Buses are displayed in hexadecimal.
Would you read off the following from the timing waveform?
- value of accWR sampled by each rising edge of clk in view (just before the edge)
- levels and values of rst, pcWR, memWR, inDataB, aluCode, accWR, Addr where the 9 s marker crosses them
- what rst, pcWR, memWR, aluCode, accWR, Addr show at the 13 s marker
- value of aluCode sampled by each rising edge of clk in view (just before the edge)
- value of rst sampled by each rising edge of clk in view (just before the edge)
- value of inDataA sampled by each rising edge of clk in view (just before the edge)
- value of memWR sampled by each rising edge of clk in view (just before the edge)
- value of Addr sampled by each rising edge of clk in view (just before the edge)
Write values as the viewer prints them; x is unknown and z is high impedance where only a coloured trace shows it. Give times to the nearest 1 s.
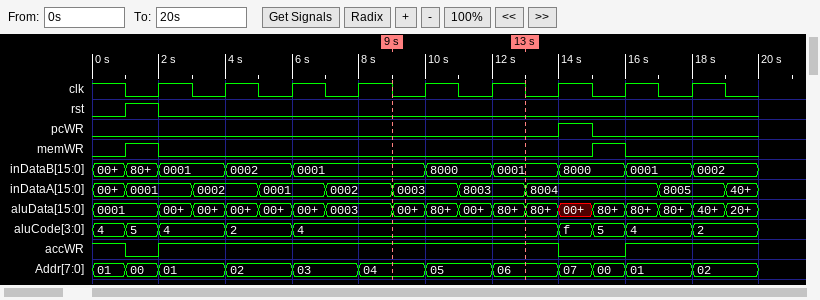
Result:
0 1 1 1 1 1 1 0 1
rst=0, pcWR=0, memWR=0, inDataB=0001, aluCode=4, accWR=1, Addr=04
rst=0, pcWR=0, memWR=0, aluCode=4, accWR=1, Addr=06
5, 4, 2, 4, 4, 4, 4, 5, 4
1 0 0 0 0 0 0 0 0
0001, 0002, 0001, 0002, 0003, 8003, 8004, 8004, 8005
1 0 0 0 0 0 0 1 0
00, 01, 02, 03, 04, 05, 06, 00, 01
